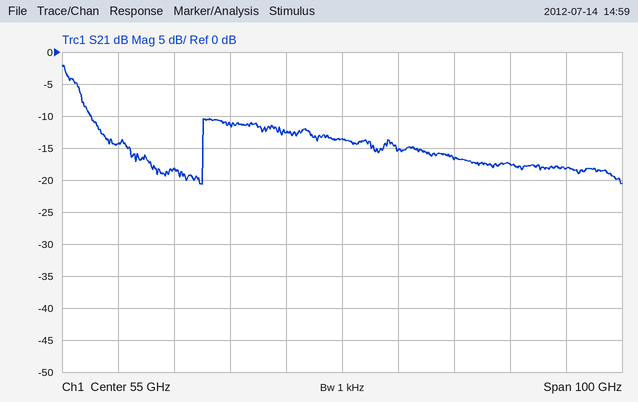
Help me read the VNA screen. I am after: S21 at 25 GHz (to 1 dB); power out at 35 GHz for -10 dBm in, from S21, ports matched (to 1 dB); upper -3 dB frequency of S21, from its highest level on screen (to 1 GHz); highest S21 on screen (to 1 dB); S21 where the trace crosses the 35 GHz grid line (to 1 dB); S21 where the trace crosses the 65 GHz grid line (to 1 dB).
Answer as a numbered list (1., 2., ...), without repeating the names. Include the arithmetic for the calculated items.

1. -18 dB
2. -10 dBm + (-11 dB) = -21 dBm
3. 8 GHz
4. -2 dB
5. -11 dB
6. -15 dB
